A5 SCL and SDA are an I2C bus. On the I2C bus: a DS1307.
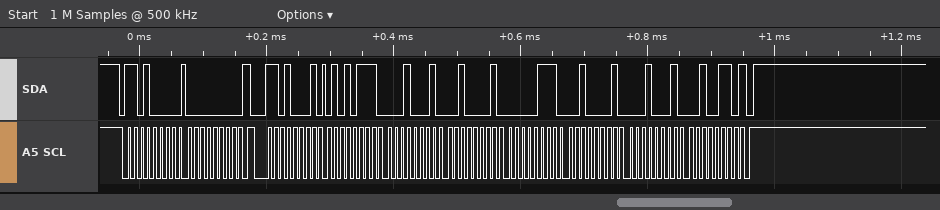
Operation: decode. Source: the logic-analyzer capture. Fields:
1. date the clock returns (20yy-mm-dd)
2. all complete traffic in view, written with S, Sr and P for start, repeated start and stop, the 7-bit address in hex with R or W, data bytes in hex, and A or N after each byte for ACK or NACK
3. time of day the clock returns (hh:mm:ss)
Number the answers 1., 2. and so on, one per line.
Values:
1. 2026-11-21
2. S 68W A 00 A Sr 68R A 57 A 11 A 21 A 07 A 21 A 11 A 26 N P
3. 21:11:57
